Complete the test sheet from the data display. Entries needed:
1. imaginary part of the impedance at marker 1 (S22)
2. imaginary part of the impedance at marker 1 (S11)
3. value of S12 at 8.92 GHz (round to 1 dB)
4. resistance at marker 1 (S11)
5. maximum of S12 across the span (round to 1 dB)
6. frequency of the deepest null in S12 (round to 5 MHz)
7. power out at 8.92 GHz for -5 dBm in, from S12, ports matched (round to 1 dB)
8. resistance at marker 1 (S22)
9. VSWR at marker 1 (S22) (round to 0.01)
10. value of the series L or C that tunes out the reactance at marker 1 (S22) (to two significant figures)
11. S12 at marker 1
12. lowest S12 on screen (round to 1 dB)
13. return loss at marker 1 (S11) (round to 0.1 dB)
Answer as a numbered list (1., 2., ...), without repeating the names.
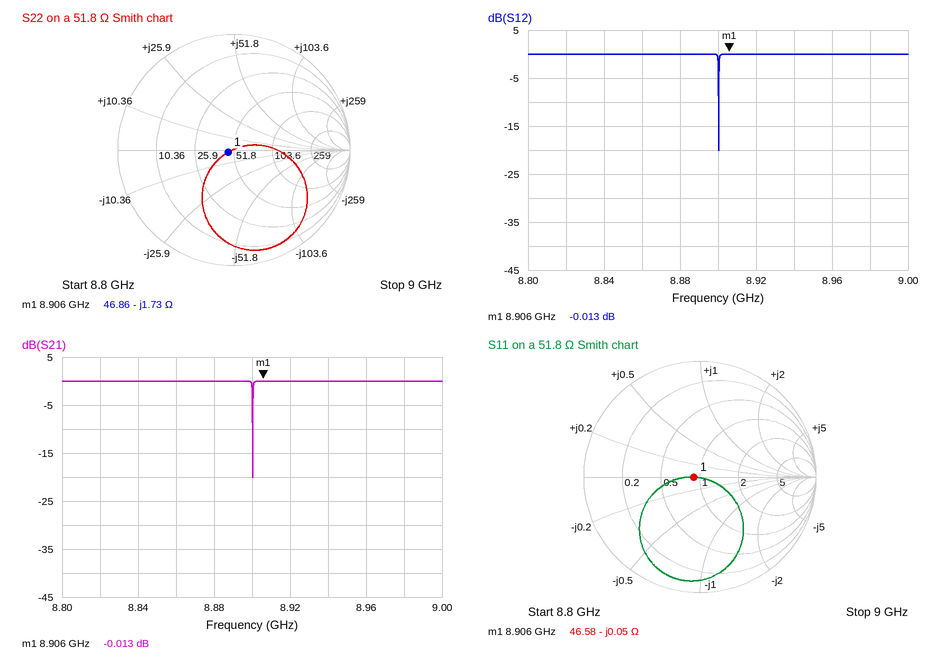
1. -1.73 Ω
2. -0.05 Ω
3. 0 dB
4. 46.58 Ω
5. 0 dB
6. 8.900 GHz
7. -5 dBm
8. 46.86 Ω
9. 1.11
10. 31 pH
11. -0.013 dB
12. -20 dB
13. 25.5 dB
